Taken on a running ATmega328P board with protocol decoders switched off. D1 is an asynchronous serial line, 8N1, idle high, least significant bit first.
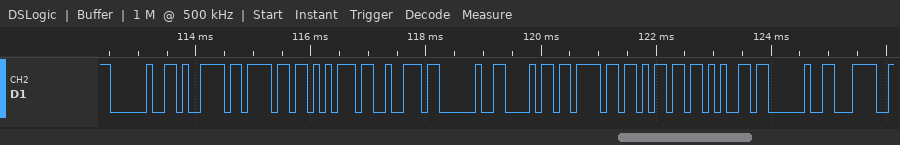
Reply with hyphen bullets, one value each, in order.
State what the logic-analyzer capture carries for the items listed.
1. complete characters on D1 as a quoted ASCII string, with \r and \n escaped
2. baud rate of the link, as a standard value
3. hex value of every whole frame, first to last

- " your home <"
- 9600 baud
- 0x20 0x79 0x6F 0x75 0x72 0x20 0x68 0x6F 0x6D 0x65 0x20 0x3C
